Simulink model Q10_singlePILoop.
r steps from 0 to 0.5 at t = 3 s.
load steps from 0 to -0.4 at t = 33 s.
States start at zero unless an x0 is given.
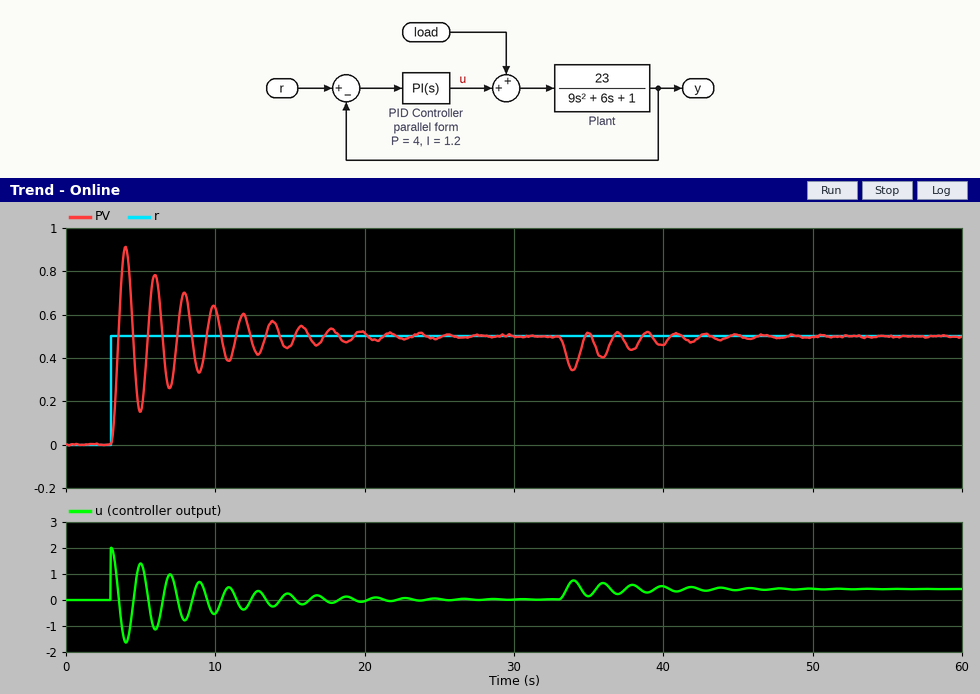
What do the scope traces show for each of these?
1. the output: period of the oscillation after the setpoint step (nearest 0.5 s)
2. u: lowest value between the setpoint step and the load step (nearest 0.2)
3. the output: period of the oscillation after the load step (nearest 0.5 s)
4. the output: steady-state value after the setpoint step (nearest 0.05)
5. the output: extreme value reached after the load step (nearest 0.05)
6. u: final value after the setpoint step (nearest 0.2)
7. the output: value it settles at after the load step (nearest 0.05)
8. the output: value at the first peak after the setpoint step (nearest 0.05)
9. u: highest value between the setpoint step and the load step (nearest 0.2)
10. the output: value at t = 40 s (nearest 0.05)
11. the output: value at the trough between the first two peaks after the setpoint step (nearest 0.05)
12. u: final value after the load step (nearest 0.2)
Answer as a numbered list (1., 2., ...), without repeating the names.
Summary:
1. 2.0 s
2. -1.6
3. 2.0 s
4. 0.50
5. 0.35
6. 0.0
7. 0.50
8. 0.90
9. 2.0
10. 0.45
11. 0.15
12. 0.4
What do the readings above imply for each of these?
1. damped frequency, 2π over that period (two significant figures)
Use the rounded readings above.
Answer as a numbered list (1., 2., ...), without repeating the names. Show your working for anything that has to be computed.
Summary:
1. 2π / 2 = 3.1 rad/s
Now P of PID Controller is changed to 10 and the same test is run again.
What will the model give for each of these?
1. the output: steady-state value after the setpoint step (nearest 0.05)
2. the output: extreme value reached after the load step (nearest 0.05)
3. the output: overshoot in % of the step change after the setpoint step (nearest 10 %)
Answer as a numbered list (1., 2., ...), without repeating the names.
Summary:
1. 0.50
2. 0.45
3. 80 %
